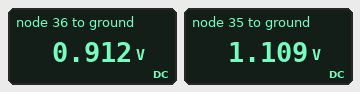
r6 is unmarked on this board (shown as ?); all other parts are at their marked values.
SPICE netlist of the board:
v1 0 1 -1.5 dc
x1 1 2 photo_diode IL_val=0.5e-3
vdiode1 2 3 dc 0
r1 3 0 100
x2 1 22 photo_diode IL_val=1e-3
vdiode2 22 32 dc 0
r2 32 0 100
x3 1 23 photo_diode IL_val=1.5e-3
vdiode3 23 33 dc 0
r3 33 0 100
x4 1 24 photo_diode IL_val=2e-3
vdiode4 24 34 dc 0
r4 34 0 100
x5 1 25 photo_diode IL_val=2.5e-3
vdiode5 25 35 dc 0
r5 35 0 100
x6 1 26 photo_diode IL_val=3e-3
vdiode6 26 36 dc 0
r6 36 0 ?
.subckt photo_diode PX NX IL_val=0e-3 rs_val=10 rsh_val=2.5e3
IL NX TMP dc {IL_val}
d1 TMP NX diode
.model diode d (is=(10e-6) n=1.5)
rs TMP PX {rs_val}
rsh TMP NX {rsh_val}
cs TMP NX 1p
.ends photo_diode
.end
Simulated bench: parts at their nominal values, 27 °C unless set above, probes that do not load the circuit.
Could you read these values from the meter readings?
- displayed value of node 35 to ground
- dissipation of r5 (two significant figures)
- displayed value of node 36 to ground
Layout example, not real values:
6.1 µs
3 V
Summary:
1.109 V
12 mW
0.912 V
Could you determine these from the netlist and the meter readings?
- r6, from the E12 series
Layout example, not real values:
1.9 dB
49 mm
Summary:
33 Ω
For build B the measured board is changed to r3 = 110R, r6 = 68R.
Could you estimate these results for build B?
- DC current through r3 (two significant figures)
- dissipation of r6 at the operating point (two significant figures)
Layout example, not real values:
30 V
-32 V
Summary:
10 mA
16 mW
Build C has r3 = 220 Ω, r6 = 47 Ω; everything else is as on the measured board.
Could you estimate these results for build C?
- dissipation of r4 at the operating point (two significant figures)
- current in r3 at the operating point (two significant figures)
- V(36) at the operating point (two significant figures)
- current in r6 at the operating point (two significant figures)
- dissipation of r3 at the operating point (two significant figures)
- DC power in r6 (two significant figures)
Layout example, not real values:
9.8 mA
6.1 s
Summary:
12 mW
5.4 mA
990 mV
21 mA
6.5 mW
21 mW
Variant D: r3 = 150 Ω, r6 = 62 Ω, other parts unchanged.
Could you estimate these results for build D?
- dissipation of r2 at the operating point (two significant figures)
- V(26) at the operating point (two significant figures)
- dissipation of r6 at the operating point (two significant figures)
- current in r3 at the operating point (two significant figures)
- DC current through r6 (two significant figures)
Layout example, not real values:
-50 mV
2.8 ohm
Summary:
12 mW
1.0 V
17 mW
7.7 mA
17 mA
